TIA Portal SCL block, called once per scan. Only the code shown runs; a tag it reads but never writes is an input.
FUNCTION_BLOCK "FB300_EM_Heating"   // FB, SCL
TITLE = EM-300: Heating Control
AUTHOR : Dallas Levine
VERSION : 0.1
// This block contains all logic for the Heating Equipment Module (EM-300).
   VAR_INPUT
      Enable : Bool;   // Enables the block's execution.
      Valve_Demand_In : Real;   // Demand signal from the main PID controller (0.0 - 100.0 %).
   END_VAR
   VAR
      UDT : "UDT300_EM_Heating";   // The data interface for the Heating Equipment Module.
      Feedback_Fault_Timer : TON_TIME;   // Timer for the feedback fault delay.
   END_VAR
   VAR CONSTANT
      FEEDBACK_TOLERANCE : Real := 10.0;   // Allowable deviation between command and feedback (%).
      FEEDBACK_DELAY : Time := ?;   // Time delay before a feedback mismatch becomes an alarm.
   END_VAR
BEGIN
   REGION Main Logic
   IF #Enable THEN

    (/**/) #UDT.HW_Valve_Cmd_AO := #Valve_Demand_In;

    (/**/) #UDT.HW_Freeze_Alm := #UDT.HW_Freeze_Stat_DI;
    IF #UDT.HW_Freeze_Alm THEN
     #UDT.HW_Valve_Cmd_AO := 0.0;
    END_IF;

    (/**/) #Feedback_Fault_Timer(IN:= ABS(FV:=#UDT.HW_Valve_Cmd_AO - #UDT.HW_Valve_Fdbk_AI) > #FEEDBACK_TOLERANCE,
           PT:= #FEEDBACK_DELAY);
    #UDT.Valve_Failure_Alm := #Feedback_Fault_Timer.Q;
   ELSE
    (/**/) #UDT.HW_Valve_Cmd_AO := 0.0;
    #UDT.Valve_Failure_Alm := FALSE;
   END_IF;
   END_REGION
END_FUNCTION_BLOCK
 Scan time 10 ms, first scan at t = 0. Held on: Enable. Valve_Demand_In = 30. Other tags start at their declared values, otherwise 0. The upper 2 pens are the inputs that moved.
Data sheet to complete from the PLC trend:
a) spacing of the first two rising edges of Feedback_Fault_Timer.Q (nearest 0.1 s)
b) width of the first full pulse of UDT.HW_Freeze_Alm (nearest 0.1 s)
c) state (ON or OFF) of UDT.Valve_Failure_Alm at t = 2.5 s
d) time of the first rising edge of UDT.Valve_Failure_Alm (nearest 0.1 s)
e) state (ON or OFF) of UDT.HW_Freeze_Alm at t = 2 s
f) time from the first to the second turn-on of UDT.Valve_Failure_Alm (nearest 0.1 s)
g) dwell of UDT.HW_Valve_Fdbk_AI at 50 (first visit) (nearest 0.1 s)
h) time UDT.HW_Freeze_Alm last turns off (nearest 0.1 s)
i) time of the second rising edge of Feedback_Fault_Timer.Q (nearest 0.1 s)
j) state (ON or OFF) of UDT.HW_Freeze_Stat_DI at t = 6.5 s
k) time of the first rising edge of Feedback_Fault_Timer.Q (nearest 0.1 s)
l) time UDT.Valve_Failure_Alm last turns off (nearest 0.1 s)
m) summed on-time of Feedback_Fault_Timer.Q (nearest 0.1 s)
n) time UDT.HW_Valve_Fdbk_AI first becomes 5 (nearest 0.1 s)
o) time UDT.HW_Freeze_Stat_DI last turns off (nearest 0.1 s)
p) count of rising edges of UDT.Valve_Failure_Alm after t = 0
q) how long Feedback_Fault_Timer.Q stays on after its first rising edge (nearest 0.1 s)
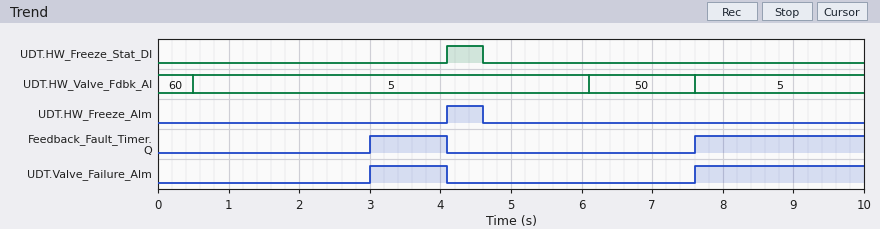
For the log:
4.6 s
0.5 s
OFF
3.0 s
OFF
4.6 s
1.5 s
4.6 s
7.6 s
OFF
3.0 s
4.1 s
3.5 s
0.5 s
4.6 s
2
1.1 s
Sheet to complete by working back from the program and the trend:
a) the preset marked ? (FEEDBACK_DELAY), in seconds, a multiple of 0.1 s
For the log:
3.0 s
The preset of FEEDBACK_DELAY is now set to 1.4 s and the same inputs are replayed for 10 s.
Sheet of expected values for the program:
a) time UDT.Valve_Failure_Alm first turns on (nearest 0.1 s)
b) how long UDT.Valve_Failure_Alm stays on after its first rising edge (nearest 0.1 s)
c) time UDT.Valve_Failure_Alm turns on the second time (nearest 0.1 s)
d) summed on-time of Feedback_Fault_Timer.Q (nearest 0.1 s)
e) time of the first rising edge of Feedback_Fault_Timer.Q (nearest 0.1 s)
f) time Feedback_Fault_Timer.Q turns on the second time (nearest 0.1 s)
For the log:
1.4 s
2.7 s
6.0 s
6.7 s
1.4 s
6.0 s
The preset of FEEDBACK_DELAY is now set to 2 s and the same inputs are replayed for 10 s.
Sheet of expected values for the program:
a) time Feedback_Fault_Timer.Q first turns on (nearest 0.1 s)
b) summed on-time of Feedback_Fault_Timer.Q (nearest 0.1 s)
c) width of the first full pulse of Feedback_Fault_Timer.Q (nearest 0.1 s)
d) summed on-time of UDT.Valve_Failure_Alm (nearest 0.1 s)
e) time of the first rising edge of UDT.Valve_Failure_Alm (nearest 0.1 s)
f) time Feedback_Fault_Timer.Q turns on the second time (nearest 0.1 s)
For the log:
2.0 s
5.5 s
2.1 s
5.5 s
2.0 s
6.6 s
